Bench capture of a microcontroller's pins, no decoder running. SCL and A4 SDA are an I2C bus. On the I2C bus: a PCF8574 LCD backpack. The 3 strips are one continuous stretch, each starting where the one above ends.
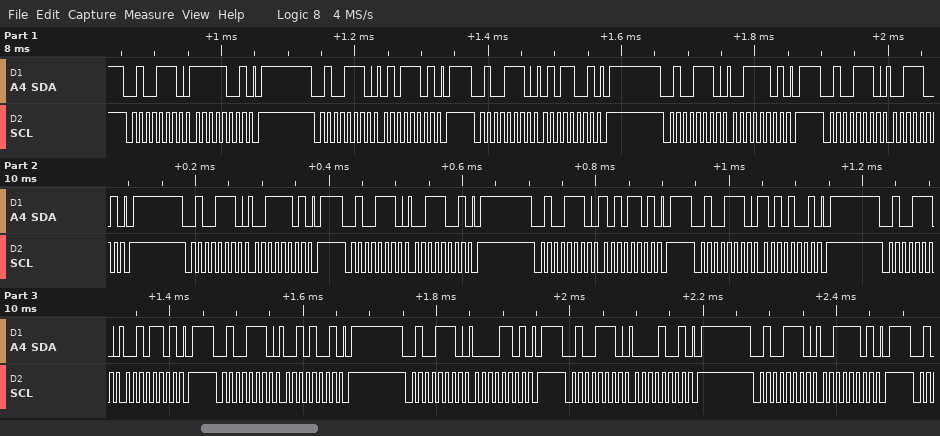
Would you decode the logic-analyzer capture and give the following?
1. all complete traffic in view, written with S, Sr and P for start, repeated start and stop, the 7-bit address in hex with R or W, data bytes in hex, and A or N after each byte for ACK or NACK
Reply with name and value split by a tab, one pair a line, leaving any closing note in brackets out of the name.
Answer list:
all complete traffic in view, written with S, Sr and P for start, repeated start and stop, the 7-bit address in hex with R or W, data bytes in hex, and A or N after each byte for ACK or NACK	S 27W A F9 A P S 27W A 5D A P S 27W A 59 A P S 27W A 3D A P S 27W A 39 A P S 27W A 3D A P S 27W A 39 A P S 27W A AD A P S 27W A A9 A P S 27W A 2D A P S 27W A 29 A P S 27W A 0D A P S 27W A 09 A P S 27W A 3D A P
